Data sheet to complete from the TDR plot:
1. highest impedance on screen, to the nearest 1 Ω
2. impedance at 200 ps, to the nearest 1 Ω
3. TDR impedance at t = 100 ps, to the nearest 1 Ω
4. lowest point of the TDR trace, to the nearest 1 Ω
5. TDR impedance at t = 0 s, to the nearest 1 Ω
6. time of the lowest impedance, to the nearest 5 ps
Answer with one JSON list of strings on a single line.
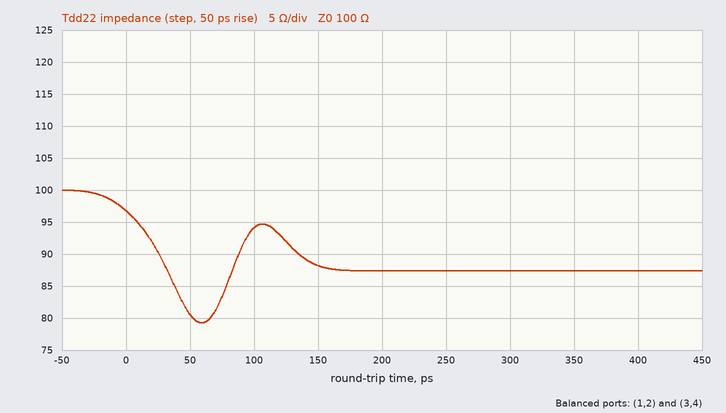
["100 Ω", "87 Ω", "94 Ω", "79 Ω", "97 Ω", "60 ps"]
